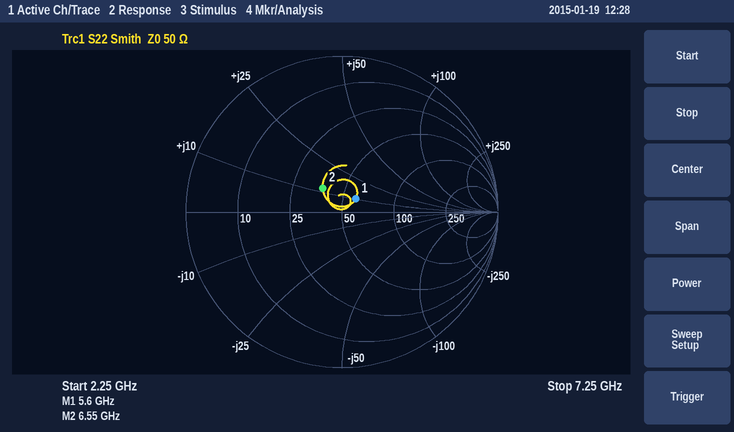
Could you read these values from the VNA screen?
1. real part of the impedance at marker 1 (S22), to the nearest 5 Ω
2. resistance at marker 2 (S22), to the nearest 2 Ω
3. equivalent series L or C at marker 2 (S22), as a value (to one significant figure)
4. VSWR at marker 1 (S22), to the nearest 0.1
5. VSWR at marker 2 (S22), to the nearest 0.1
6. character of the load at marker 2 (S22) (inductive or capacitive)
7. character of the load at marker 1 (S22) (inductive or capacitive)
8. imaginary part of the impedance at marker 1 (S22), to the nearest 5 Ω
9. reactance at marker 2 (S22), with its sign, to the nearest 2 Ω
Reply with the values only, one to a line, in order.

60 Ω
38 Ω
300 pH
1.3
1.5
inductive
inductive
+10 Ω
+12 Ω
